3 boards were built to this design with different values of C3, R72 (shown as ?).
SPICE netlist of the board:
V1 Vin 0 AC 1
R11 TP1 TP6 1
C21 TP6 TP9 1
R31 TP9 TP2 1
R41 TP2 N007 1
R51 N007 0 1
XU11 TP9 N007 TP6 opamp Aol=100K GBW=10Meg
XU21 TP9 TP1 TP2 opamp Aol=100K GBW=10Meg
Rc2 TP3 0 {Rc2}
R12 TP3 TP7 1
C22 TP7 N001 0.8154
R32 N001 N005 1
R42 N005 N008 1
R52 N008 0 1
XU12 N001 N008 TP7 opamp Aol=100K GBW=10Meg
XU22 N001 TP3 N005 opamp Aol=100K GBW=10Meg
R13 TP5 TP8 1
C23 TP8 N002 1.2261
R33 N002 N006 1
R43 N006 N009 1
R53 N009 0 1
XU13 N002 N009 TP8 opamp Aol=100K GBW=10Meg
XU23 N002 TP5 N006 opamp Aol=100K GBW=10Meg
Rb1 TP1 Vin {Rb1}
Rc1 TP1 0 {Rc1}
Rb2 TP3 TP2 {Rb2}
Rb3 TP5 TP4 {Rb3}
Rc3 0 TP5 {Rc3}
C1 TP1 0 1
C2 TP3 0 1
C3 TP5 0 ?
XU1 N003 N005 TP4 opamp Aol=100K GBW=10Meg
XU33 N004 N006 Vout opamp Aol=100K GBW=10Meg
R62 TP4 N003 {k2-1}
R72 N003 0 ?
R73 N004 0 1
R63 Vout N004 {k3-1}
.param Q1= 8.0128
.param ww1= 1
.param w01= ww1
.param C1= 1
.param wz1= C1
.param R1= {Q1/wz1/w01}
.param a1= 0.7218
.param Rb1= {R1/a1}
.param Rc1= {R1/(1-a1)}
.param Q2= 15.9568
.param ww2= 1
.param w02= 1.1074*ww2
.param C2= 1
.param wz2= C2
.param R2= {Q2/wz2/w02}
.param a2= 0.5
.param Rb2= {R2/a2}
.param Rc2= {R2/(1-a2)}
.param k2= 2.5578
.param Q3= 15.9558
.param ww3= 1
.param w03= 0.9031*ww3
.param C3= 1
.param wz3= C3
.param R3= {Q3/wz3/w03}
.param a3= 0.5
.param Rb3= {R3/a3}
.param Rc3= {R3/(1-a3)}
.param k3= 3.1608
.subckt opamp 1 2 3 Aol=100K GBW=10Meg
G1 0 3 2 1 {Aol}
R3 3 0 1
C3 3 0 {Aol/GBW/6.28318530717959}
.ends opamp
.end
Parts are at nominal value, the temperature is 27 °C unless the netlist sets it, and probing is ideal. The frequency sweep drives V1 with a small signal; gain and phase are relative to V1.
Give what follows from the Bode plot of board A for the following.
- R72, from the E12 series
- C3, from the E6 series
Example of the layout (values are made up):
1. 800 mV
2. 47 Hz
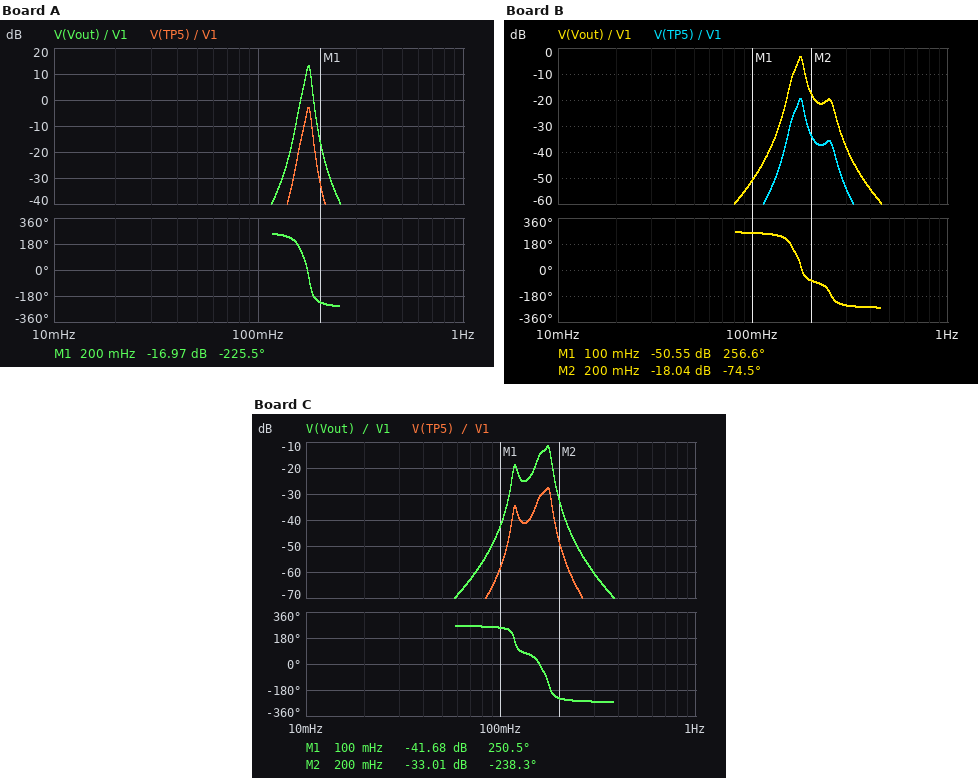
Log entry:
1. 1.8 Ω
2. 680 mF
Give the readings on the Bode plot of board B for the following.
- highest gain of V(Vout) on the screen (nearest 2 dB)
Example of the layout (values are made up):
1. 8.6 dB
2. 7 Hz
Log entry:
1. -4 dB
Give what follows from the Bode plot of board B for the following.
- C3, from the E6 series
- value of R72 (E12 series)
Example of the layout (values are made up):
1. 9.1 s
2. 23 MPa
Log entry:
1. 330 mF
2. 1.8 Ω
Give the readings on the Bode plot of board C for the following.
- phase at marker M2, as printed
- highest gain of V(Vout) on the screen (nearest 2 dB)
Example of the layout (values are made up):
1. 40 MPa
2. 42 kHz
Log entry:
1. -238.3 deg
2. -12 dB
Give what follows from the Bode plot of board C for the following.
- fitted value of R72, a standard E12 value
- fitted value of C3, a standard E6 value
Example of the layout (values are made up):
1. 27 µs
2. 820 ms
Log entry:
1. 2.2 Ω
2. 1.5 F
